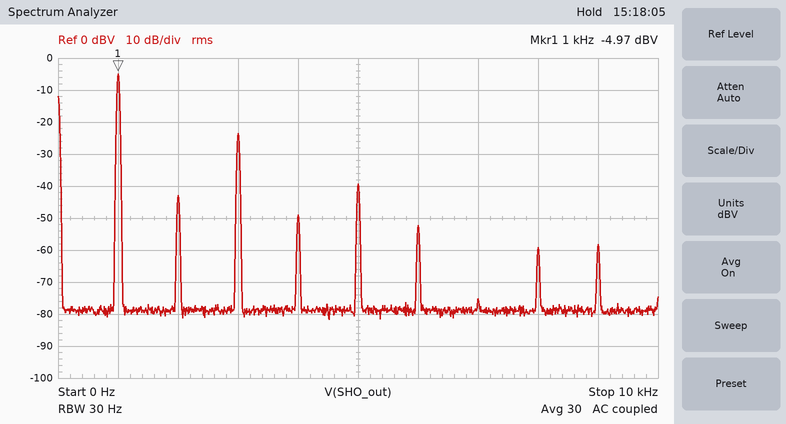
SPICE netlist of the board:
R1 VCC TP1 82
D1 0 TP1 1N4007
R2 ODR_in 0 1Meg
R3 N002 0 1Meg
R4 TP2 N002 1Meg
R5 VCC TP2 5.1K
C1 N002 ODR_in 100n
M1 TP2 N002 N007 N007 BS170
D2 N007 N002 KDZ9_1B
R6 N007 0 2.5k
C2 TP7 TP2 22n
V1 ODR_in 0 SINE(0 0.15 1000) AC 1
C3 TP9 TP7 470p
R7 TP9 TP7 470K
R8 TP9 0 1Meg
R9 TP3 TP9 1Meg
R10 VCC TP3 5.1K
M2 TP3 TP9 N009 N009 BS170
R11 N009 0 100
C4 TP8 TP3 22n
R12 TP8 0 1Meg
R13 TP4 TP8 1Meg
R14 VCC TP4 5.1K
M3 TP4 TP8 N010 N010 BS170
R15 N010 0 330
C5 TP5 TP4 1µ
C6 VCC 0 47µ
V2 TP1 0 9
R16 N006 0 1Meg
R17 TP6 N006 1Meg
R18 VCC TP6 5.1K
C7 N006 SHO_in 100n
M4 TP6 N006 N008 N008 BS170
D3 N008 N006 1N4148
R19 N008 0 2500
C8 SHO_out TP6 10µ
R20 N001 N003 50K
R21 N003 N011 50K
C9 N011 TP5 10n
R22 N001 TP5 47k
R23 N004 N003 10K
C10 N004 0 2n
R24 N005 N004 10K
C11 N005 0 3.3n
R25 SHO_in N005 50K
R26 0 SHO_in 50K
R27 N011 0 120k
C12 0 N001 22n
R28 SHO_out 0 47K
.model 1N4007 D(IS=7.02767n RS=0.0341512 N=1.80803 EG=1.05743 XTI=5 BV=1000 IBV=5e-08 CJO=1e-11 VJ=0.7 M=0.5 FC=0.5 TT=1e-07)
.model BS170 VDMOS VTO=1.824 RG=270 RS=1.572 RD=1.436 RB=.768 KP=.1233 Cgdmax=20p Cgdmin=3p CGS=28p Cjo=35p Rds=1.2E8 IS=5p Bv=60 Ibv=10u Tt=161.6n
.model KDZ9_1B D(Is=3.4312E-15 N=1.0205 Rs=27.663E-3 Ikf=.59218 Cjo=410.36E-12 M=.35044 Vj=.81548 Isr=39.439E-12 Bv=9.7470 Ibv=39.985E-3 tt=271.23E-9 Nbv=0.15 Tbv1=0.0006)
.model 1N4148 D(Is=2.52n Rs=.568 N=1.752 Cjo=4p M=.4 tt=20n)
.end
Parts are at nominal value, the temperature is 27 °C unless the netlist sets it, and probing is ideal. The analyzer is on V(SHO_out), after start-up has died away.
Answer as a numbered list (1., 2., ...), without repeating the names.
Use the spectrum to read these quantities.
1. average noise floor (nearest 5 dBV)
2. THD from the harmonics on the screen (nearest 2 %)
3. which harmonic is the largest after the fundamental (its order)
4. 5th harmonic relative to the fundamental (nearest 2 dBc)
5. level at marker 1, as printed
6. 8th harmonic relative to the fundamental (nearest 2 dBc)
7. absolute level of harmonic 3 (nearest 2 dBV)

1. -80 dBV
2. 12 %
3. 3
4. -34 dBc
5. -4.97 dBV
6. -54 dBc
7. -24 dBV
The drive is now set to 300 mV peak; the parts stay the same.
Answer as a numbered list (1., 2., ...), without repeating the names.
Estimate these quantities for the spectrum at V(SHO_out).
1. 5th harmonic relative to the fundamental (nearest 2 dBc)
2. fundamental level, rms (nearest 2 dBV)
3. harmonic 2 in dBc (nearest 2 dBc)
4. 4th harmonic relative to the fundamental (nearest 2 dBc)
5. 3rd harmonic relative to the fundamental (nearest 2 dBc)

1. -26 dBc
2. -4 dBV
3. -36 dBc
4. -46 dBc
5. -16 dBc
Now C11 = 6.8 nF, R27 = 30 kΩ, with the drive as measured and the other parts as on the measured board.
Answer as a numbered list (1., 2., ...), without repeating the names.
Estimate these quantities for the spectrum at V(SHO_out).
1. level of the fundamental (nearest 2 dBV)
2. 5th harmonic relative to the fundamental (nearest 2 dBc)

1. -10 dBV
2. -36 dBc
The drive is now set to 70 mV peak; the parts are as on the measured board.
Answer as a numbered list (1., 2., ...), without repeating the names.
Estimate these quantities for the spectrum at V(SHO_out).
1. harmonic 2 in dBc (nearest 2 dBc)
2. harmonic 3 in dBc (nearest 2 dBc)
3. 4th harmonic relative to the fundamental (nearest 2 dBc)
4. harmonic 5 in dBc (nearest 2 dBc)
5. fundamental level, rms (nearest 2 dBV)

1. -28 dBc
2. -36 dBc
3. -54 dBc
4. -50 dBc
5. -6 dBV
